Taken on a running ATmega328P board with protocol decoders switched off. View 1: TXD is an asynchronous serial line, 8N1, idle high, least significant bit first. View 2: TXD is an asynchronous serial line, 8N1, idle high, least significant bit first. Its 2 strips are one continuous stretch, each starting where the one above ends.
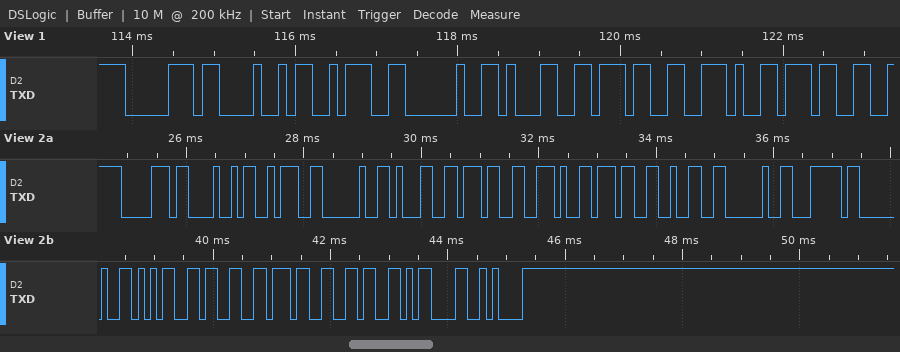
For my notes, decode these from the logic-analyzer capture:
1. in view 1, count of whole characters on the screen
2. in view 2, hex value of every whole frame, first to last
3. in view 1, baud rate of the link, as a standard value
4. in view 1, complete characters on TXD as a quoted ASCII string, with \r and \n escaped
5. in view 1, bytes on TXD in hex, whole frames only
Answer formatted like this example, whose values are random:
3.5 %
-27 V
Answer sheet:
8
70 48 3A 20 31 37 2E 37 32 20 7C 20 35 33 37 36 0D 0A
9600 baud
"pH: 17.7"
0x70 0x48 0x3A 0x20 0x31 0x37 0x2E 0x37
